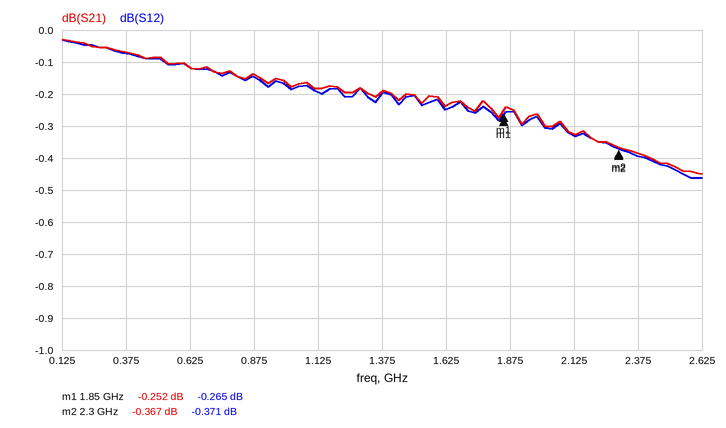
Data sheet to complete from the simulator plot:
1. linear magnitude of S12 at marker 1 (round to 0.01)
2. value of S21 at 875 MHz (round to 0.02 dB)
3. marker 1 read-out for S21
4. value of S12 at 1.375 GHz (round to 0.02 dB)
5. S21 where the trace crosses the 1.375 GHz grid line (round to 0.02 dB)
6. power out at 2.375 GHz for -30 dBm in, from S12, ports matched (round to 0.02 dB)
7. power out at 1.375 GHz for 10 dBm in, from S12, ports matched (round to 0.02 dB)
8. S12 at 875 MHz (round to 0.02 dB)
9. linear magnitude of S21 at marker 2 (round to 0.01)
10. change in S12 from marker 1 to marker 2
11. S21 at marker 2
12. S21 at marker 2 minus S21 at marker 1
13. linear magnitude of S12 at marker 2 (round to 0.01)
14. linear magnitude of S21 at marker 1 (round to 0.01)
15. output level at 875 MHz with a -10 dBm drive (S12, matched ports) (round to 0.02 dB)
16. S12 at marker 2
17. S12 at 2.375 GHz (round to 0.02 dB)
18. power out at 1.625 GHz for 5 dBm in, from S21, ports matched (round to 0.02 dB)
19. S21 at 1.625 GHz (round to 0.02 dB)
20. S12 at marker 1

0.97
-0.14 dB
-0.252 dB
-0.20 dB
-0.20 dB
-30.40 dBm
9.80 dBm
-0.14 dB
0.96
-0.106 dB
-0.367 dB
-0.115 dB
0.96
0.97
-10.14 dBm
-0.371 dB
-0.40 dB
4.76 dBm
-0.24 dB
-0.265 dB
